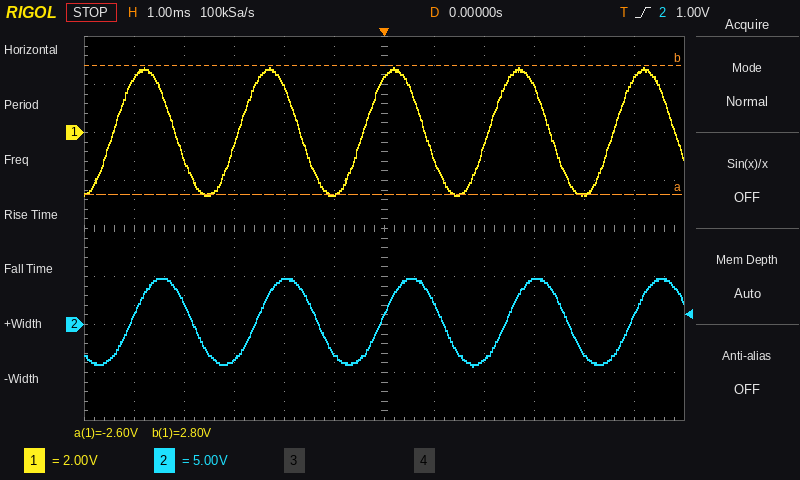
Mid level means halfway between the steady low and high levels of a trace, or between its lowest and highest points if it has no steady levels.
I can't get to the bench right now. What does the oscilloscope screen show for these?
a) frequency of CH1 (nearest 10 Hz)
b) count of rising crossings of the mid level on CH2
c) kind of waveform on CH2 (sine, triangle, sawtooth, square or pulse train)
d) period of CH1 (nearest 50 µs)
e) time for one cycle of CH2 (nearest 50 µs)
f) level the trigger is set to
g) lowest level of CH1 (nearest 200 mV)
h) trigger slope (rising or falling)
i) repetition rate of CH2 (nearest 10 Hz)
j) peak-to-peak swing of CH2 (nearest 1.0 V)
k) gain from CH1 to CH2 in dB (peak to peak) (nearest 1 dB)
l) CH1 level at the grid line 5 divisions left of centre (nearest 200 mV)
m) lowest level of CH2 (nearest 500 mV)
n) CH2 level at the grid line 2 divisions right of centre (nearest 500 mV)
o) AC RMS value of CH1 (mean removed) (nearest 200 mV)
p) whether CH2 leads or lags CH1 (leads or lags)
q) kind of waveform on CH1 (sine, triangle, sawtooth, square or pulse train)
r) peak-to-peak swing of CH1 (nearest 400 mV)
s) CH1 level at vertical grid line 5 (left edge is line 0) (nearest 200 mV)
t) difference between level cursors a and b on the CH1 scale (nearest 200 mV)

400 Hz
5
sine
2.50 ms
2.50 ms
1.00 V
-2.6 V
rising
400 Hz
9.0 V
5 dB
2.2 V
-4.5 V
-3.5 V
1.8 V
lags
sine
5.2 V
-2.6 V
5.4 V
